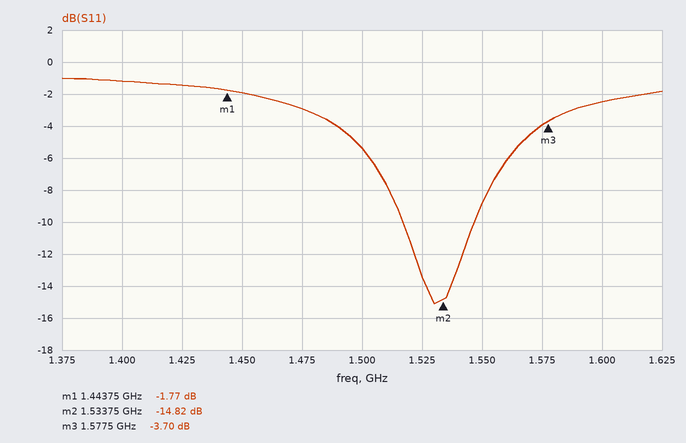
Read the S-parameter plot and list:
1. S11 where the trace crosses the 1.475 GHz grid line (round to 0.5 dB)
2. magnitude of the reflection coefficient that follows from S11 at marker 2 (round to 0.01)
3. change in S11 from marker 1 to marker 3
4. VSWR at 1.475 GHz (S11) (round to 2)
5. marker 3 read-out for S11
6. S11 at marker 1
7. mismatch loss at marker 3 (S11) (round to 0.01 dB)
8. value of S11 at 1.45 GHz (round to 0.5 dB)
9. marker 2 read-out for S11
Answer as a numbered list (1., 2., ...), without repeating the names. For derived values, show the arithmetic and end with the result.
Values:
1. -3.0 dB
2. 10^(-14.82/20) ≈ 0.18
3. -3.7 − (-1.77) = -1.93 dB
4. |Γ| = 10^(-3/20) = 0.7079; VSWR = (1 + 0.7079)/(1 − 0.7079) ≈ 6
5. -3.70 dB
6. -1.77 dB
7. −10 log10(1 − 10^(-3.7/10)) ≈ 2.42 dB
8. -2.0 dB
9. -14.82 dB
